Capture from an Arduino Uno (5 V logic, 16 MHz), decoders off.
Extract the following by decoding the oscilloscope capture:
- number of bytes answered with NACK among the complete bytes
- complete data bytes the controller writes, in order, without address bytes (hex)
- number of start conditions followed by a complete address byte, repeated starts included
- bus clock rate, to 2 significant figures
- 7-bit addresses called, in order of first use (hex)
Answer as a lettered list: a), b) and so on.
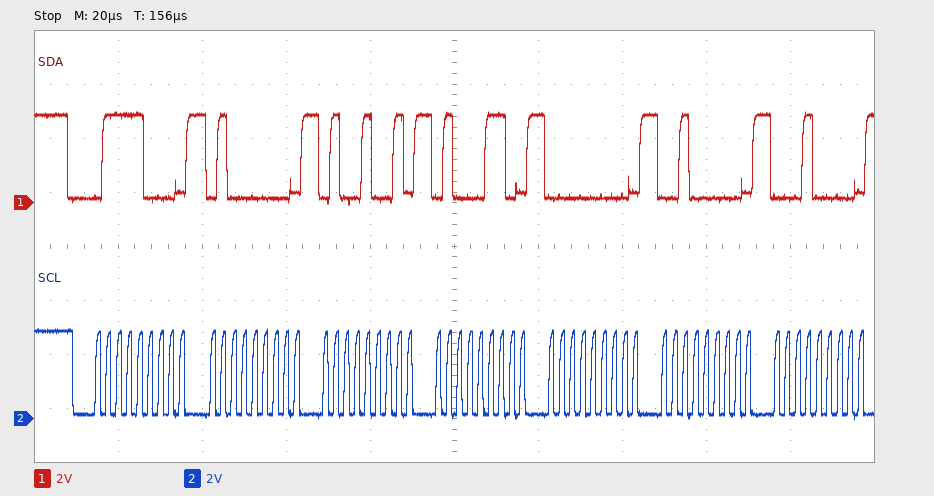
a) 0
b) 40 49 46 00 20 10
c) 1
d) 400 kHz
e) 0x3C
